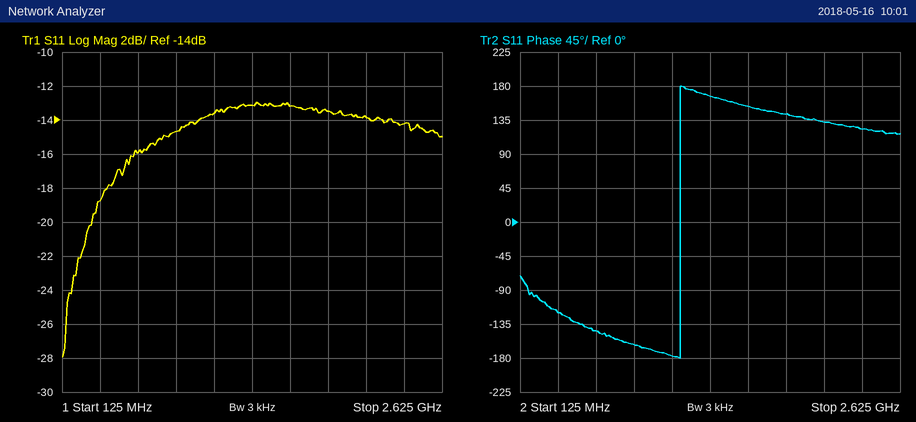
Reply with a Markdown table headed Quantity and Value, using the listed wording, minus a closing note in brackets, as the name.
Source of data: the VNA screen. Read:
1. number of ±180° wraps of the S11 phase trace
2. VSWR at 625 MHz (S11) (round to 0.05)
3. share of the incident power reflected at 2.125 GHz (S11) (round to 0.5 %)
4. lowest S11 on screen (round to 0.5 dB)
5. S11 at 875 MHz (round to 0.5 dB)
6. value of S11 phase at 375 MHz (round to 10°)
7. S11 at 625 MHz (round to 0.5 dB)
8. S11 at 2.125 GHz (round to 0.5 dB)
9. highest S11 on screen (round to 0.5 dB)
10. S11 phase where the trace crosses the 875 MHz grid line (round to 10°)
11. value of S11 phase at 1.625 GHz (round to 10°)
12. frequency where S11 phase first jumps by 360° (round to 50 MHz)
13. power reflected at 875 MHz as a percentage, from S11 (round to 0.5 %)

| Quantity | Value |
|---|---|
| number of ±180° wraps of the S11 phase trace | 1 |
| VSWR at 625 MHz (S11) | 1.40 |
| share of the incident power reflected at 2.125 GHz (S11) | 4.0 % |
| lowest S11 on screen | -28.0 dB |
| S11 at 875 MHz | -14.5 dB |
| value of S11 phase at 375 MHz | -120° |
| S11 at 625 MHz | -16.0 dB |
| S11 at 2.125 GHz | -14.0 dB |
| highest S11 on screen | -13.0 dB |
| S11 phase where the trace crosses the 875 MHz grid line | -160° |
| value of S11 phase at 1.625 GHz | 150° |
| frequency where S11 phase first jumps by 360° | 1.20 GHz |
| power reflected at 875 MHz as a percentage, from S11 | 3.5 % |
